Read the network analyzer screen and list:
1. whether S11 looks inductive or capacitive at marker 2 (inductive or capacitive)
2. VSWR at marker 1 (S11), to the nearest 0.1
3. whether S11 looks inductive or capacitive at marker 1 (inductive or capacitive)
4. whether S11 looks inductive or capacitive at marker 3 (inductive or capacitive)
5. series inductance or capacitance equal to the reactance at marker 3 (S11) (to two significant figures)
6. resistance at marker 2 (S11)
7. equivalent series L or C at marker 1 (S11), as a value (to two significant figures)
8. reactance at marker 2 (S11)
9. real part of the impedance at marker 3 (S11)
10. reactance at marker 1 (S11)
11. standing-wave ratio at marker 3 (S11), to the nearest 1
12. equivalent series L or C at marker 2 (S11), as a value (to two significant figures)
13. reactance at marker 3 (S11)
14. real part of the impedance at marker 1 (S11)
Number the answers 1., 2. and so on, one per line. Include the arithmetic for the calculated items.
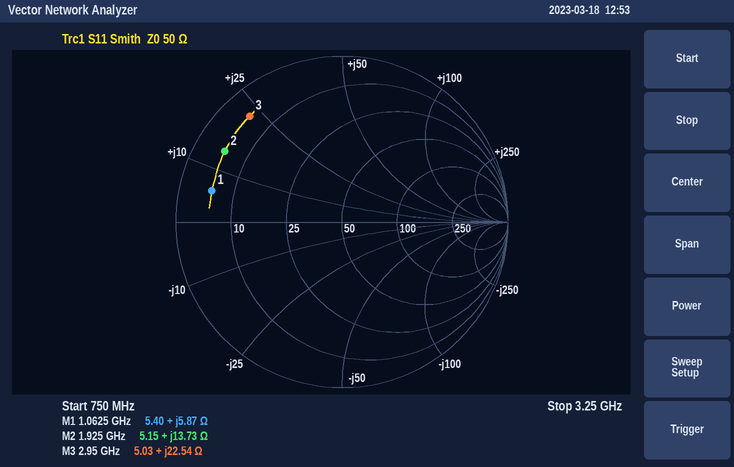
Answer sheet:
1. inductive
2. 9.4
3. inductive
4. inductive
5. L = 22.54 Ω/(2π × 2.95 GHz) ≈ 1.2 nH
6. 5.15 Ω
7. L = 5.87 Ω/(2π × 1.0625 GHz) ≈ 879 pH, so 880 pH to two significant figures
8. +13.73 Ω
9. 5.03 Ω
10. +5.87 Ω
11. 12
12. L = 13.73 Ω/(2π × 1.925 GHz) ≈ 1.1 nH
13. +22.54 Ω
14. 5.40 Ω
